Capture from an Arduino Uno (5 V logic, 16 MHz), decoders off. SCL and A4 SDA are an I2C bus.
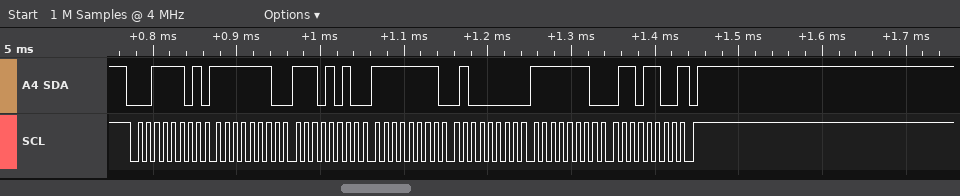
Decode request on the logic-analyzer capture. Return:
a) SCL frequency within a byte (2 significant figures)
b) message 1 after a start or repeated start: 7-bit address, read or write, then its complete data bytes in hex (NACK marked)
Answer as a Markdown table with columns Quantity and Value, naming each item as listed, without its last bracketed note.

| Quantity | Value |
|---|---|
| SCL frequency within a byte | 100 kHz |
| message 1 after a start or repeated start: 7-bit address, read or write, then its complete data bytes in hex | 0x1E read: FE EA FF 40 FE 6C NACK |
